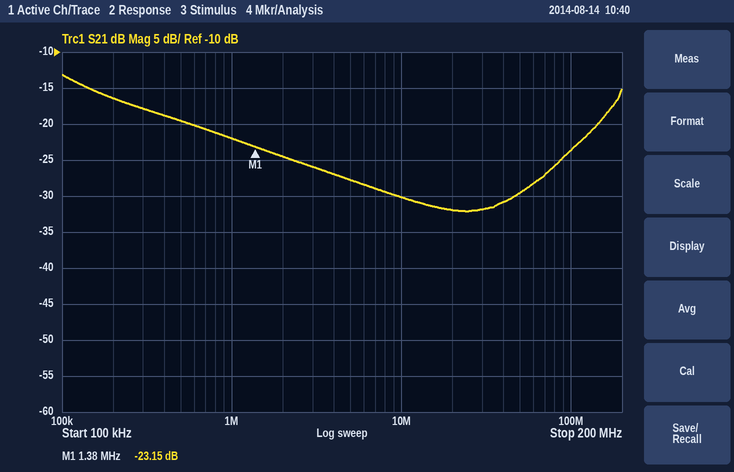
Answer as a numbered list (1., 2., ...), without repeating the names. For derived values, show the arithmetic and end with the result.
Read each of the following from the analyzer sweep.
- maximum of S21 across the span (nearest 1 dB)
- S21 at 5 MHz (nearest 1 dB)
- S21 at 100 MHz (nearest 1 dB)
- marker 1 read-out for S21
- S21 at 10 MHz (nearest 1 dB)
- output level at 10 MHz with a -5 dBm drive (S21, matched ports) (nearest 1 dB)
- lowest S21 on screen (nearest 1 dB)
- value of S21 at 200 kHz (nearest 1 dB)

1. -13 dB
2. -28 dB
3. -24 dB
4. -23.15 dB
5. -30 dB
6. -5 dBm + (-30 dB) = -35 dBm
7. -32 dB
8. -16 dB
